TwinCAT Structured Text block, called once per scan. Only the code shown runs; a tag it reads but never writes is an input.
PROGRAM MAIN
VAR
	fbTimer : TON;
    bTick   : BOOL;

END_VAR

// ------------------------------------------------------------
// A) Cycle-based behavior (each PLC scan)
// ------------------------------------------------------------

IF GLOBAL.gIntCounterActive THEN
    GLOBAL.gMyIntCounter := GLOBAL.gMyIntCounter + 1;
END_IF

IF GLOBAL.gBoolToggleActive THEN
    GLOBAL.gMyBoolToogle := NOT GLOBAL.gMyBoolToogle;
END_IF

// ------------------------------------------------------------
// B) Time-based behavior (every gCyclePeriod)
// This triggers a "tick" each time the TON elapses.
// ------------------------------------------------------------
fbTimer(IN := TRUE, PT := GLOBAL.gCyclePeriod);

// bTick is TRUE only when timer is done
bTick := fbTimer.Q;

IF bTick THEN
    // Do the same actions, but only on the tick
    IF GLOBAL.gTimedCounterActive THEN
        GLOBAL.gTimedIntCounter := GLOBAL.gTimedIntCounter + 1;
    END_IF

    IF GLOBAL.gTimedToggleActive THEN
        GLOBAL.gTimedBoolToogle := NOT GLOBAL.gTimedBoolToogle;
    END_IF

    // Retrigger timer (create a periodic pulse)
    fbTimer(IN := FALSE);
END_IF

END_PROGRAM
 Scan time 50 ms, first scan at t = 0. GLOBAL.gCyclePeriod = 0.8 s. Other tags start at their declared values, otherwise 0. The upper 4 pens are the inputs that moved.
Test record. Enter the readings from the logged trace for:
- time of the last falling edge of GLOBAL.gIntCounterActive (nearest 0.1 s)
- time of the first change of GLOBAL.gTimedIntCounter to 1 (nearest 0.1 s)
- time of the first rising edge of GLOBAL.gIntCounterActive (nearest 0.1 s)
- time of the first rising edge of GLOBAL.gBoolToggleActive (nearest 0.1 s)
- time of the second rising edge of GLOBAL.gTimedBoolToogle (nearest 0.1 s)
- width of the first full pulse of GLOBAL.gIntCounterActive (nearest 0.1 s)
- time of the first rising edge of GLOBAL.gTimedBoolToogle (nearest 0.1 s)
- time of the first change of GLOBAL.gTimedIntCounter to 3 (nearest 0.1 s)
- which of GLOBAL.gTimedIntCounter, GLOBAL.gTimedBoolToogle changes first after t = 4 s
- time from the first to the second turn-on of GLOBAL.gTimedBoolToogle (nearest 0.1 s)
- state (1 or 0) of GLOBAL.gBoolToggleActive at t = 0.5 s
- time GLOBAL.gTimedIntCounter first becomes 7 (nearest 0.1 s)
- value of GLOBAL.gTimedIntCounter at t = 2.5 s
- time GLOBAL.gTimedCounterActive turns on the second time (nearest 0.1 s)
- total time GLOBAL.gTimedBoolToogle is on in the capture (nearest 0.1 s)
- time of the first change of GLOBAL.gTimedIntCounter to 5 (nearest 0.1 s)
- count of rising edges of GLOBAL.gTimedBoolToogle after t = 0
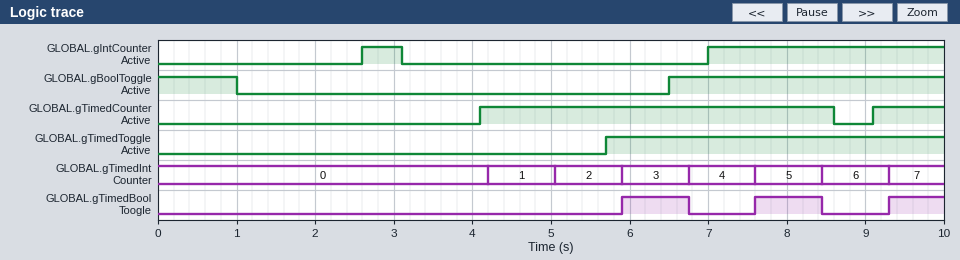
3.1 s
4.2 s
2.6 s
6.5 s
7.6 s
0.5 s
5.9 s
5.9 s
GLOBAL.gTimedIntCounter
1.7 s
1
9.3 s
0
9.1 s
2.4 s
7.6 s
3
